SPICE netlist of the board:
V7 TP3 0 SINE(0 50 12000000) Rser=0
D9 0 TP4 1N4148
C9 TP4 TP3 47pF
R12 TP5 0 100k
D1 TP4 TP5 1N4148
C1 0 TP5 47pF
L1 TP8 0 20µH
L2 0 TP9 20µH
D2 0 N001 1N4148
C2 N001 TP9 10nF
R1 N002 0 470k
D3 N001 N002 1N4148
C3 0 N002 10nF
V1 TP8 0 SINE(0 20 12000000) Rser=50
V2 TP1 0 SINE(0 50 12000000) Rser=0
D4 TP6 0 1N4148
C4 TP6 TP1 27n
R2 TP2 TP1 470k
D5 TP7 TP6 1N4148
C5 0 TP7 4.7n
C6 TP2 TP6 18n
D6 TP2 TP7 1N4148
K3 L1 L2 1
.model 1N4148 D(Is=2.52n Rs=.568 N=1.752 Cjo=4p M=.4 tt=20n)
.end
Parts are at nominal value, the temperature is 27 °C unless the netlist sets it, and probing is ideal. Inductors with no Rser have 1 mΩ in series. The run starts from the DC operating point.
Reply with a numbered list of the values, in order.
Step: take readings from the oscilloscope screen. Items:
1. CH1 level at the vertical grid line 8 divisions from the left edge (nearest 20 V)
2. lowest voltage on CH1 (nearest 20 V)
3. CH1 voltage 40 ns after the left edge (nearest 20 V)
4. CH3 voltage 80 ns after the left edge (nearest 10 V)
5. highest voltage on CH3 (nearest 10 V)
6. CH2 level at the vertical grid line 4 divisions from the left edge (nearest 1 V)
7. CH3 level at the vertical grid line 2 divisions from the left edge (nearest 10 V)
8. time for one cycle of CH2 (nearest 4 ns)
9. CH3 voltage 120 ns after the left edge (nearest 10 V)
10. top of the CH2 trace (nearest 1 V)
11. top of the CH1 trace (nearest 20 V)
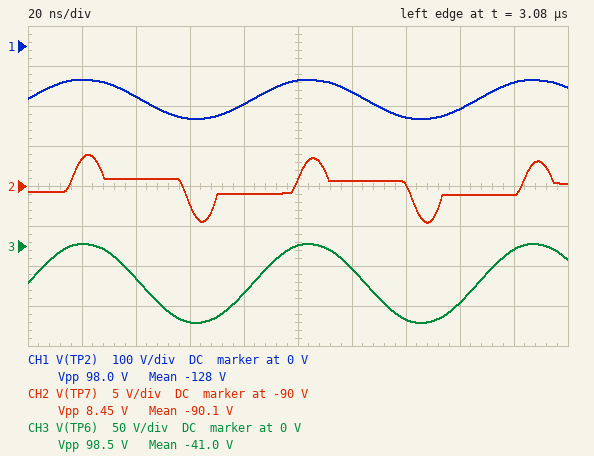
1. -160 V
2. -180 V
3. -120 V
4. -60 V
5. 0 V
6. -91 V
7. -40 V
8. 84 ns
9. -30 V
10. -86 V
11. -80 V
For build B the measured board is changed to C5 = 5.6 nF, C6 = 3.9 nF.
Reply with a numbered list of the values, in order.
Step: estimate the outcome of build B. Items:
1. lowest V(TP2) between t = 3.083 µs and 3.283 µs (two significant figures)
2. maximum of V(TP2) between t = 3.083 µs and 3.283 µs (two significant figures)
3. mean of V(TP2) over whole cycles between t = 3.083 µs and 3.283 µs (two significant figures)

1. -190 V
2. -94 V
3. -140 V
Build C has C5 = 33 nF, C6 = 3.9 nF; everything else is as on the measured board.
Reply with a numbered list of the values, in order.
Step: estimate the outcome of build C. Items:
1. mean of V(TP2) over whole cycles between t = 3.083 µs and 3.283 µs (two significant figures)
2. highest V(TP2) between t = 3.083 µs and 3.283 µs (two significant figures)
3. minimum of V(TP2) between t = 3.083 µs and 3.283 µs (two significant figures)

1. -140 V
2. -90 V
3. -190 V
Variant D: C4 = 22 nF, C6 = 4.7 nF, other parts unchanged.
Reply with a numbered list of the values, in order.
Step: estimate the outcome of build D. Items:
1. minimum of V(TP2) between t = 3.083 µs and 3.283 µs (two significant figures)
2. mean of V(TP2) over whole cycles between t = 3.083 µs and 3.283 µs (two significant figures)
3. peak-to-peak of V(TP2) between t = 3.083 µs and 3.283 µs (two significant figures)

1. -190 V
2. -140 V
3. 99 V
